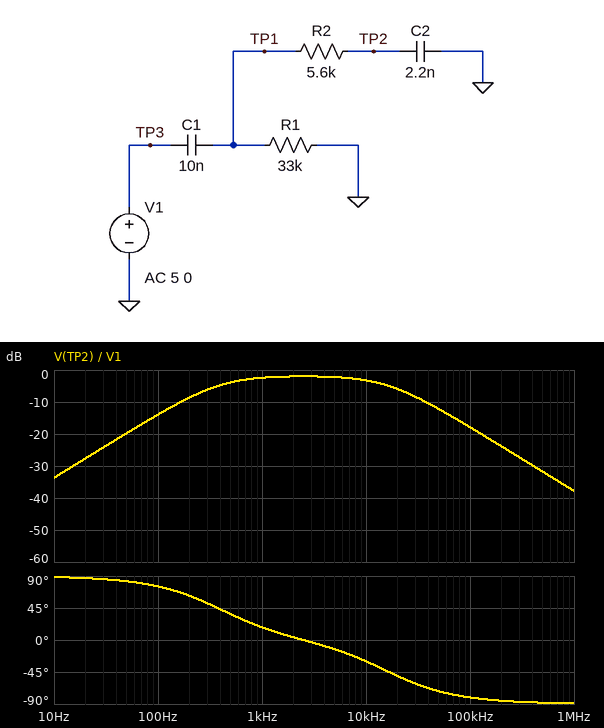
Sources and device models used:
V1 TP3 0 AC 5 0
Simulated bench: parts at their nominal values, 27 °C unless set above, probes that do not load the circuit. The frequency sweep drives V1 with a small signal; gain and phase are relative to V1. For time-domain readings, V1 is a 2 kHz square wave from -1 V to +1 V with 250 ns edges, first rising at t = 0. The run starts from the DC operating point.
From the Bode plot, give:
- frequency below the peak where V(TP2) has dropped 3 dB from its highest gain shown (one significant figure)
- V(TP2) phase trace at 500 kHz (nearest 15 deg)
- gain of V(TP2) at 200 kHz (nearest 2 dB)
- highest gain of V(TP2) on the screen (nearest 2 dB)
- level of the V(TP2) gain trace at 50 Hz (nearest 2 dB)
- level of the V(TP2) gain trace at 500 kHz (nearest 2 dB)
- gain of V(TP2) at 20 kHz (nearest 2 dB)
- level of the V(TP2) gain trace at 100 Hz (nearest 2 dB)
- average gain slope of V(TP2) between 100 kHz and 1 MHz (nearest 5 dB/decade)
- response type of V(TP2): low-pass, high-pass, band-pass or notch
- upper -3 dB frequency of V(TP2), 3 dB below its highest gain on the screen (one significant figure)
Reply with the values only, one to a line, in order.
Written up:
400 Hz
-90 deg
-24 dB
-2 dB
-20 dB
-32 dB
-6 dB
-14 dB
-20 dB/decade
band-pass
20 kHz
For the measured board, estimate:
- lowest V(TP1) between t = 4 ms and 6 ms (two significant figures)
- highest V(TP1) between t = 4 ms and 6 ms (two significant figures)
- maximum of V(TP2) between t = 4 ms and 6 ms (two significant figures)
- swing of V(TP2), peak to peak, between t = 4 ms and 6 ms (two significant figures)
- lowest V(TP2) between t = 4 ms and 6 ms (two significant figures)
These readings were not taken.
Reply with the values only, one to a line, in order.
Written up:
-1.4 V
1.4 V
950 mV
1.9 V
-950 mV
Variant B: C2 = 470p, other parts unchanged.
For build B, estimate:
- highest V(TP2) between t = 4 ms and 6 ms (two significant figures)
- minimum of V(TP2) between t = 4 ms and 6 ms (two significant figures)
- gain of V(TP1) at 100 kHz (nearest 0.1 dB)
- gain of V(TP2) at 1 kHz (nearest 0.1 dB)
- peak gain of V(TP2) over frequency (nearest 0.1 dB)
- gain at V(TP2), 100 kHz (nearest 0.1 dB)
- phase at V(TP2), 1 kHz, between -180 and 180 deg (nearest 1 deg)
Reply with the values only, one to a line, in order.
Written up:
1.2 V
-1.2 V
-0.1 dB
-1.2 dB
-0.5 dB
-5.8 dB
24 deg
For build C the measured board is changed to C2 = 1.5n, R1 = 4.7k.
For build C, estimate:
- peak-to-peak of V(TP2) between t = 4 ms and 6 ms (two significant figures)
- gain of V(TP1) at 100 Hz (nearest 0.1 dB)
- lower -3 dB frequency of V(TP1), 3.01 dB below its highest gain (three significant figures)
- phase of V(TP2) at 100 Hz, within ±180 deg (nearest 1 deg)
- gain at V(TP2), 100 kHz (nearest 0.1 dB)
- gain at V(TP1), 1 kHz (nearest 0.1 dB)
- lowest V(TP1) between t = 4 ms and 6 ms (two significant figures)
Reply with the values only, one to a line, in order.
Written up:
2.5 V
-30.6 dB
4.23 kHz
88 deg
-14.7 dB
-11.1 dB
-2.0 V
